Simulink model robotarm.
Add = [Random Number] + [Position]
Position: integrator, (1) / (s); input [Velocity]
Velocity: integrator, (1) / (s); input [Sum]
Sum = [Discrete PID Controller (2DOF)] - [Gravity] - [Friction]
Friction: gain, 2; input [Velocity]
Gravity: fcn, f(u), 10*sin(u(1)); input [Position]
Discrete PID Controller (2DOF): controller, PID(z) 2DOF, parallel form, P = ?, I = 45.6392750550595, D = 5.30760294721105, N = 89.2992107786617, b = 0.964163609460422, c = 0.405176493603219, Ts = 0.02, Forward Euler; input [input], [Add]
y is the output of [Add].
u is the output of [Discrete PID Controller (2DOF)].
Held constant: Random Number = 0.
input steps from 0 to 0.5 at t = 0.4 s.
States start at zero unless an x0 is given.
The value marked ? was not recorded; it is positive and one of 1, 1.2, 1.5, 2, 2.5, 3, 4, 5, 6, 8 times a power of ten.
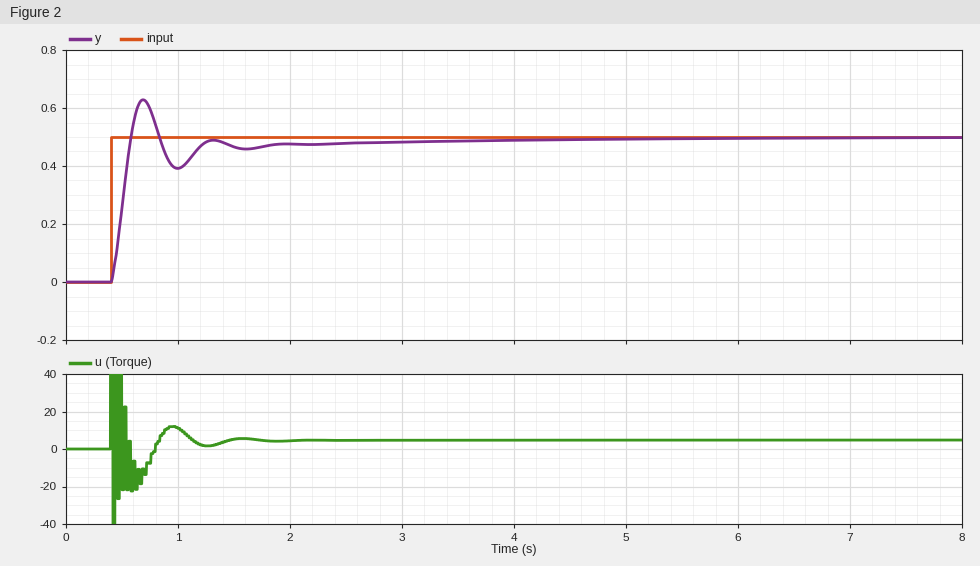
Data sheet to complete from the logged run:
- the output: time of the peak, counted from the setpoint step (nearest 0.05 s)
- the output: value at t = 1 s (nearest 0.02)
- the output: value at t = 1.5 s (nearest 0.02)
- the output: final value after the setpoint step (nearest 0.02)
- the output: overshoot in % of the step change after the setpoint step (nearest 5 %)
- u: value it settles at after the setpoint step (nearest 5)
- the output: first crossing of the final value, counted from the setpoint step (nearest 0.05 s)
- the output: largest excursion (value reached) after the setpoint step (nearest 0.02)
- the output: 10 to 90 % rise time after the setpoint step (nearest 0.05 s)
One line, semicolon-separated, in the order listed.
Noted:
0.30 s; 0.40; 0.46; 0.50; 25 %; 5; 0.20 s; 0.62; 0.15 s
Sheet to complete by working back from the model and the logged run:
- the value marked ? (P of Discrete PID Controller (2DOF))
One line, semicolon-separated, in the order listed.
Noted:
100
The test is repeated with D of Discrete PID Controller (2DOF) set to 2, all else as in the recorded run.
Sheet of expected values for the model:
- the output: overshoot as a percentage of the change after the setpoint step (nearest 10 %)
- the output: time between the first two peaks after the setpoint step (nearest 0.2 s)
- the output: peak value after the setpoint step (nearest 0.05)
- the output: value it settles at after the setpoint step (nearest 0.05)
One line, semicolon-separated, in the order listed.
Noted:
50 %; 0.6 s; 0.75; 0.50
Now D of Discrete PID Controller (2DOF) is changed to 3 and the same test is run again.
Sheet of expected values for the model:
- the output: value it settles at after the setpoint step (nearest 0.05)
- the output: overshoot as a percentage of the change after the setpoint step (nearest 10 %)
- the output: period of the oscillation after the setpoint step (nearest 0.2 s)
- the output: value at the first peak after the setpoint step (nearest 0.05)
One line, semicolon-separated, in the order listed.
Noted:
0.50; 40 %; 0.6 s; 0.70
